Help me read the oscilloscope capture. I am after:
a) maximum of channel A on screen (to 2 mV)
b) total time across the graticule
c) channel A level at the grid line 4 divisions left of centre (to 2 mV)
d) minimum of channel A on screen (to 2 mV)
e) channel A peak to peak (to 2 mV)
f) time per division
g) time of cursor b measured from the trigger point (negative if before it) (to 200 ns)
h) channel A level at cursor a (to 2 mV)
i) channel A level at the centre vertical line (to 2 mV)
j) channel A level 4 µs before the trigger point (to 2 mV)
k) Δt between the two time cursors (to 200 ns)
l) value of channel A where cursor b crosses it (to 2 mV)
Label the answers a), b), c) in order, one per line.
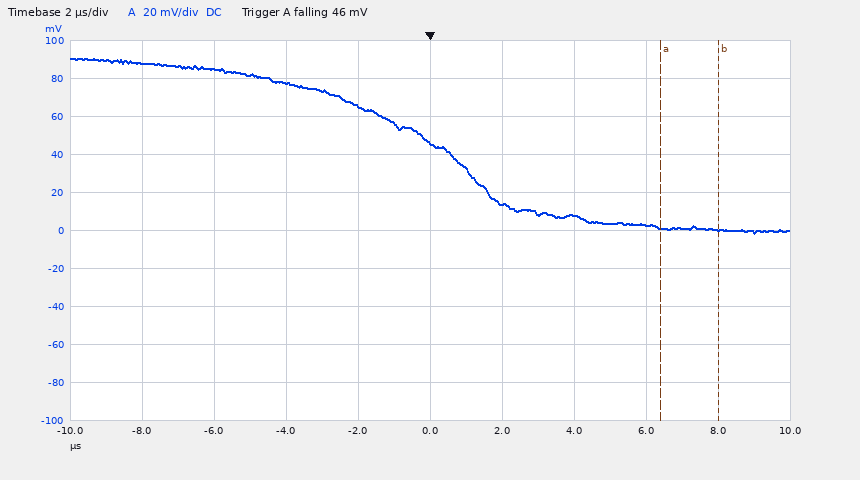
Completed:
a) 90 mV
b) 20 µs
c) 88 mV
d) -2 mV
e) 92 mV
f) 2 µs
g) +8.0 µs
h) 2 mV
i) 46 mV
j) 78 mV
k) 1.6 µs
l) 0 mV
